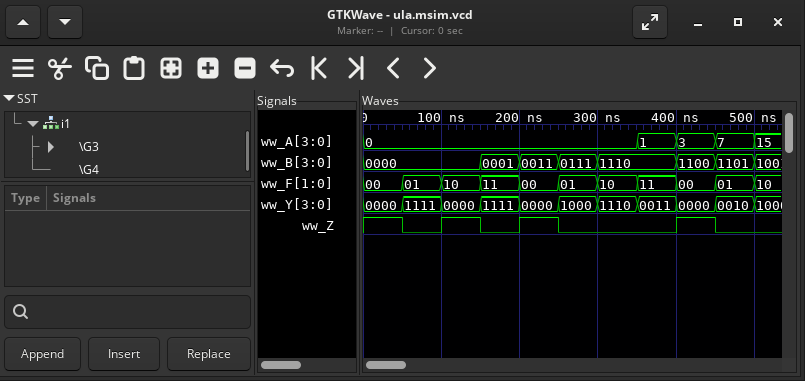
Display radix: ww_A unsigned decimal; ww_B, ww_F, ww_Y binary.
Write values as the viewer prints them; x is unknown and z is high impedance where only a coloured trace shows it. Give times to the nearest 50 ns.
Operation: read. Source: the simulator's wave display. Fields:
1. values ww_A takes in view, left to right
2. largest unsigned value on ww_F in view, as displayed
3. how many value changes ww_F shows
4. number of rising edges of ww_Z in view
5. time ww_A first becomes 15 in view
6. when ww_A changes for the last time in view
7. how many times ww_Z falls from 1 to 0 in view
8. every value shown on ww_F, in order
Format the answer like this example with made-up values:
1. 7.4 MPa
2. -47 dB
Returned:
1. 0, 1, 3, 7, 15
2. 11
3. 10
4. 3
5. 500 ns
6. 500 ns
7. 4
8. 00, 01, 10, 11, 00, 01, 10, 11, 00, 01, 10
